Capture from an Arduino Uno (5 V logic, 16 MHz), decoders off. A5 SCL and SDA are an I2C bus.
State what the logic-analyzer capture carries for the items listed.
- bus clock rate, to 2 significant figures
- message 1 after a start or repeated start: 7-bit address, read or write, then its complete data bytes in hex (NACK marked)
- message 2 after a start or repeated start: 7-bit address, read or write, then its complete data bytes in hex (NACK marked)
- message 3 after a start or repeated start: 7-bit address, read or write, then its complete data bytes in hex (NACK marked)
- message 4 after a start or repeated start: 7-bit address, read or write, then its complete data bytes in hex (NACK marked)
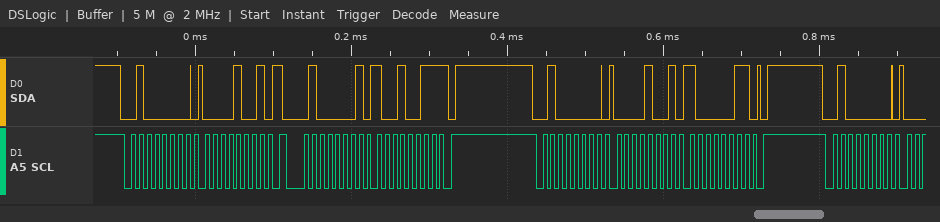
100 kHz
0x20 write: 09
0x20 read: 93 NACK
0x20 write: 09 83
0x20 write
